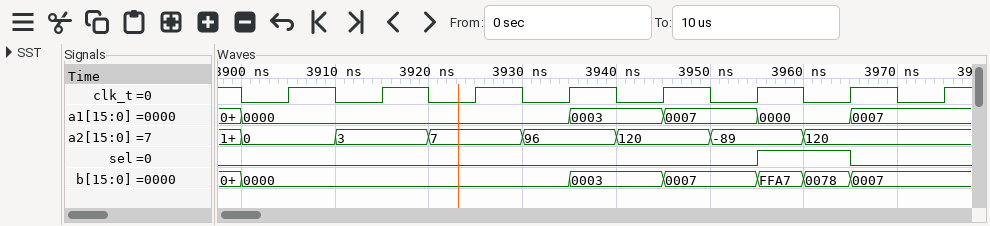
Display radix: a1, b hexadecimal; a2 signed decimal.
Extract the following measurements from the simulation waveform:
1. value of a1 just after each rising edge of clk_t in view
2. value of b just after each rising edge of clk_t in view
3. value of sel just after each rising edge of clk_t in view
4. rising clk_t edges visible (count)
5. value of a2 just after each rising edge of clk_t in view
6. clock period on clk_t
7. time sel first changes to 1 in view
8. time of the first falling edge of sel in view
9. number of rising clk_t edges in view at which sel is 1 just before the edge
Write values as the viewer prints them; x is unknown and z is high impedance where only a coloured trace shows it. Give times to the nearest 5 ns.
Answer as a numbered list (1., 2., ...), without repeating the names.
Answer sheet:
1. 0000, 0000, 0000, 0003, 0007, 0000, 0007, 0007
2. 0000, 0000, 0000, 0003, 0007, FFA7, 0007, 0007
3. 0 0 0 0 0 1 0 0
4. 8
5. 0, 3, 7, 96, 120, -89, 120, 120
6. 10 ns
7. 3955 ns
8. 3965 ns
9. 1
